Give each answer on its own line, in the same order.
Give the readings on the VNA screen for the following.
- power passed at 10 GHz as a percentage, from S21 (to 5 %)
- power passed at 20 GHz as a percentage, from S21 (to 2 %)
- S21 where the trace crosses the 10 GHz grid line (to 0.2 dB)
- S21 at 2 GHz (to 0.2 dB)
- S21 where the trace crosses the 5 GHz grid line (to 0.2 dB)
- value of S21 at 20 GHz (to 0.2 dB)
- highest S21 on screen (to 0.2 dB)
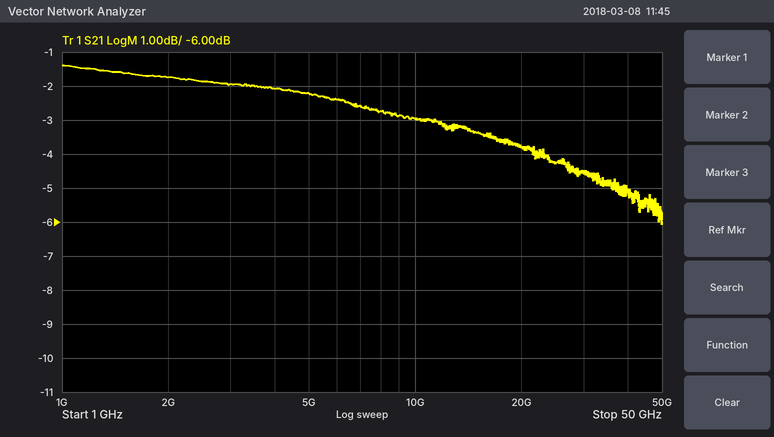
50 %
42 %
-3.0 dB
-1.8 dB
-2.2 dB
-3.8 dB
-1.4 dB
